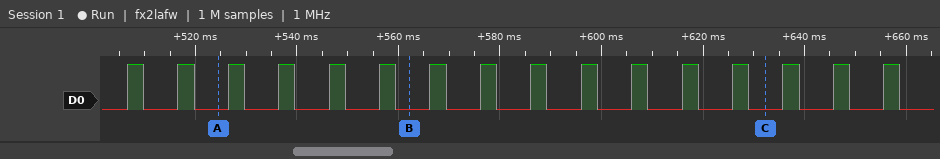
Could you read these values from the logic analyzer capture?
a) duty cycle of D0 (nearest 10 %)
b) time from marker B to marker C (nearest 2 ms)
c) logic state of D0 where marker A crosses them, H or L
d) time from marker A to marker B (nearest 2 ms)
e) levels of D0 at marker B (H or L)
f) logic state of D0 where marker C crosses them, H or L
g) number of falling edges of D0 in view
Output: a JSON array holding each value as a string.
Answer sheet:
["30 %", "70 ms", "D0=L", "38 ms", "D0=L", "D0=L", "16"]
